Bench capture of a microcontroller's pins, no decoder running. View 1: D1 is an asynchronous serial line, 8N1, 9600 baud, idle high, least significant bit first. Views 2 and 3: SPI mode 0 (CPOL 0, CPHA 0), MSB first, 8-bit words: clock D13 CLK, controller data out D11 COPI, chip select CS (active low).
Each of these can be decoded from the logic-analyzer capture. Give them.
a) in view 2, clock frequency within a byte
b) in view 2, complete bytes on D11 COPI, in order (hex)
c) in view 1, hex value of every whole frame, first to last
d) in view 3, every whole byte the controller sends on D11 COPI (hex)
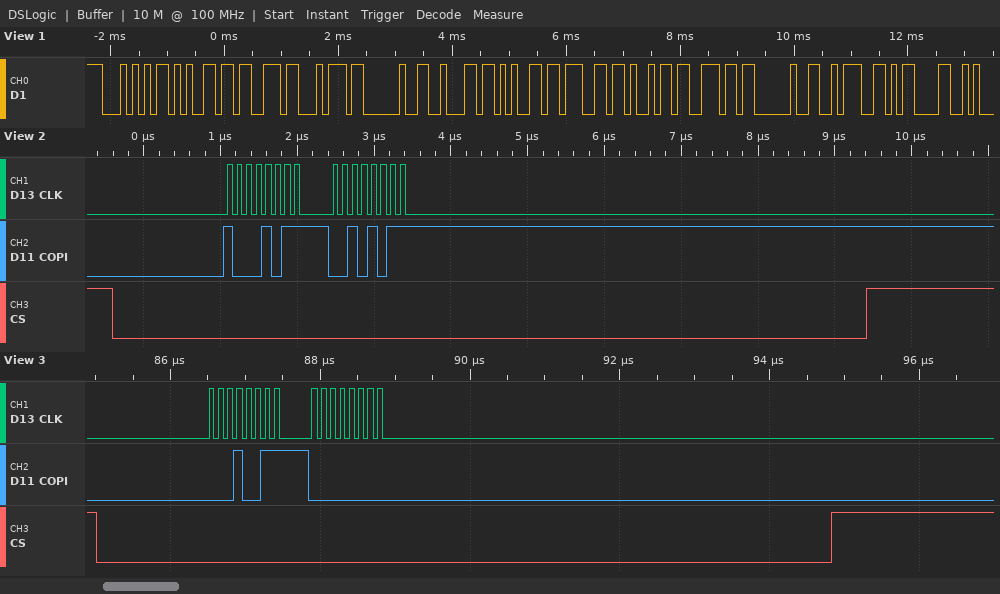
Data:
8 MHz
8B 2B
0x54 0x65 0x73 0x74 0x20 0x62 0x65 0x67 0x69 0x6E 0x20 0x3A 0x0D
13 00
